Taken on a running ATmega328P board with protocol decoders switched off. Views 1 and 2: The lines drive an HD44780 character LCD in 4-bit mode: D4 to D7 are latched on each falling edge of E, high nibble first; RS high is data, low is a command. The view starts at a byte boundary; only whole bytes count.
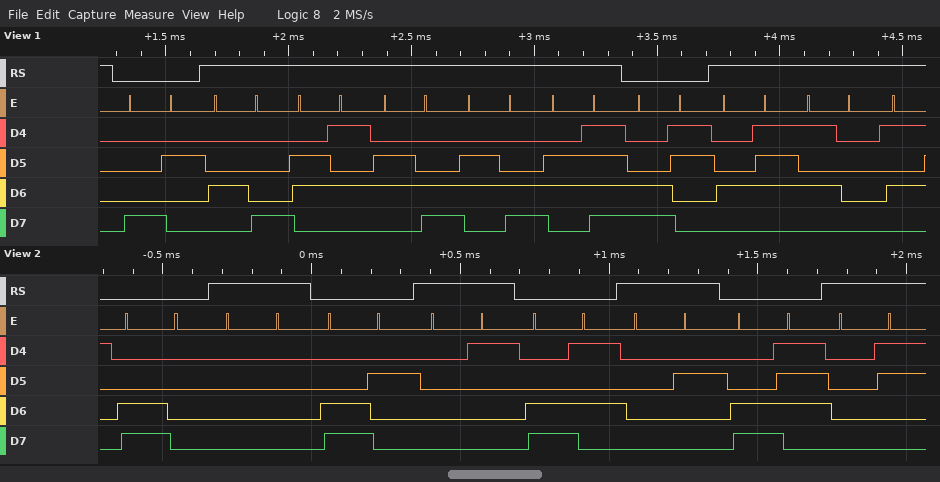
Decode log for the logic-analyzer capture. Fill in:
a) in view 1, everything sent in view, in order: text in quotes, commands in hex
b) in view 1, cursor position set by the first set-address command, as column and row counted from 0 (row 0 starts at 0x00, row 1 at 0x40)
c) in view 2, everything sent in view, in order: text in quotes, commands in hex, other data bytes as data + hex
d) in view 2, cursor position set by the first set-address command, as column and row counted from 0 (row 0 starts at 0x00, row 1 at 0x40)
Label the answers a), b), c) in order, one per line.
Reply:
a) 0x82 "Hello" 0xC3 "GP"
b) column 2, row 0
c) 0xC0 data 00 0xC2 data 01 0xC5 data 02 0xC7 data 03
d) column 0, row 1
